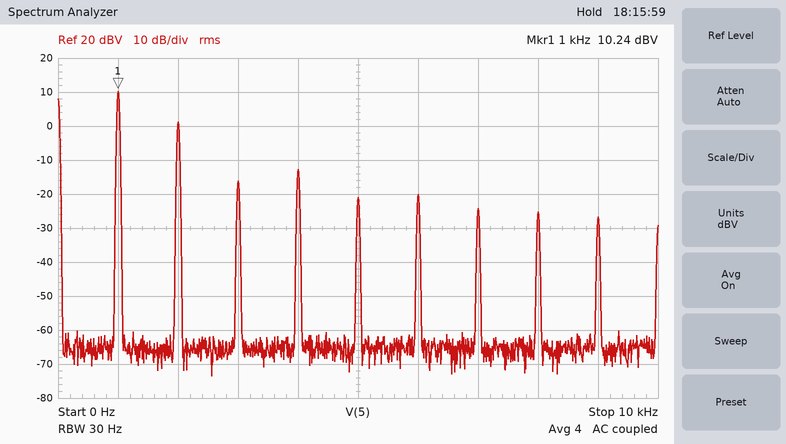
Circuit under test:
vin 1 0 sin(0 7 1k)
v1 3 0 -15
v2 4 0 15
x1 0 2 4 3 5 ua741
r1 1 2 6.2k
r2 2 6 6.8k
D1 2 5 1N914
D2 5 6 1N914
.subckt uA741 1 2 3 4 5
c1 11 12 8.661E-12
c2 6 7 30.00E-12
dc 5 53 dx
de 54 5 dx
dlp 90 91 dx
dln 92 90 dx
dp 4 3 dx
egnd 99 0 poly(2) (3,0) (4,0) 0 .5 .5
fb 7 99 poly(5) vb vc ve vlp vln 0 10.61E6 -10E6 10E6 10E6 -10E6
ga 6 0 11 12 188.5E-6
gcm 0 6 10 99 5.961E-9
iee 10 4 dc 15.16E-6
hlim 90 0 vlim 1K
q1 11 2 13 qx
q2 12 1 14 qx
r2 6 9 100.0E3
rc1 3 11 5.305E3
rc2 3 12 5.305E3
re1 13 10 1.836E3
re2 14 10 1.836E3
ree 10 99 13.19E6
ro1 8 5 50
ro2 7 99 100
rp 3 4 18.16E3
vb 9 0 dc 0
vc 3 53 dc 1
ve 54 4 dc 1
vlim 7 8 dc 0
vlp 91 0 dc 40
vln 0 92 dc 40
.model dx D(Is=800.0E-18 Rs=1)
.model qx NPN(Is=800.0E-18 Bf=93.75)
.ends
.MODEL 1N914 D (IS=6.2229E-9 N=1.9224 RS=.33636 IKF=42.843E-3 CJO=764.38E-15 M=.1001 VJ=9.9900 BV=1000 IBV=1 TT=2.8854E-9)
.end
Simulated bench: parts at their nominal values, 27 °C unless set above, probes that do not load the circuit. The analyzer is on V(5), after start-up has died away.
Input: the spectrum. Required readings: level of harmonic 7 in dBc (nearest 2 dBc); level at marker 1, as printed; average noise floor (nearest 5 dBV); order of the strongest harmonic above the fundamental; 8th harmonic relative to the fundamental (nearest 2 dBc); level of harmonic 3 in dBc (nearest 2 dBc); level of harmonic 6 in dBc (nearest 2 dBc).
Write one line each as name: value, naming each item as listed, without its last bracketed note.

level of harmonic 7 in dBc: -34 dBc
level at marker 1, as printed: 10.24 dBV
average noise floor: -65 dBV
order of the strongest harmonic above the fundamental: 2
8th harmonic relative to the fundamental: -36 dBc
level of harmonic 3 in dBc: -26 dBc
level of harmonic 6 in dBc: -30 dBc
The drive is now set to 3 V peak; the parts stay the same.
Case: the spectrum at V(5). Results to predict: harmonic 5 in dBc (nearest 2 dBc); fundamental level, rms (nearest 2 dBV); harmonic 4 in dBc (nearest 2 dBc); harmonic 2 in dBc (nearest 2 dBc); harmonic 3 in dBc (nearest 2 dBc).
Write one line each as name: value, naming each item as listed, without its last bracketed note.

harmonic 5 in dBc: -26 dBc
fundamental level, rms: 4 dBV
harmonic 4 in dBc: -24 dBc
harmonic 2 in dBc: -10 dBc
harmonic 3 in dBc: -22 dBc
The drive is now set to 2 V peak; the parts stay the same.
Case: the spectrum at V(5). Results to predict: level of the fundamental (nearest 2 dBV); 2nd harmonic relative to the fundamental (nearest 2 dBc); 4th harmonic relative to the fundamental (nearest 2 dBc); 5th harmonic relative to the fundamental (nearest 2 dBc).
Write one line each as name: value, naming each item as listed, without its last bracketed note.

level of the fundamental: 2 dBV
2nd harmonic relative to the fundamental: -12 dBc
4th harmonic relative to the fundamental: -26 dBc
5th harmonic relative to the fundamental: -24 dBc
